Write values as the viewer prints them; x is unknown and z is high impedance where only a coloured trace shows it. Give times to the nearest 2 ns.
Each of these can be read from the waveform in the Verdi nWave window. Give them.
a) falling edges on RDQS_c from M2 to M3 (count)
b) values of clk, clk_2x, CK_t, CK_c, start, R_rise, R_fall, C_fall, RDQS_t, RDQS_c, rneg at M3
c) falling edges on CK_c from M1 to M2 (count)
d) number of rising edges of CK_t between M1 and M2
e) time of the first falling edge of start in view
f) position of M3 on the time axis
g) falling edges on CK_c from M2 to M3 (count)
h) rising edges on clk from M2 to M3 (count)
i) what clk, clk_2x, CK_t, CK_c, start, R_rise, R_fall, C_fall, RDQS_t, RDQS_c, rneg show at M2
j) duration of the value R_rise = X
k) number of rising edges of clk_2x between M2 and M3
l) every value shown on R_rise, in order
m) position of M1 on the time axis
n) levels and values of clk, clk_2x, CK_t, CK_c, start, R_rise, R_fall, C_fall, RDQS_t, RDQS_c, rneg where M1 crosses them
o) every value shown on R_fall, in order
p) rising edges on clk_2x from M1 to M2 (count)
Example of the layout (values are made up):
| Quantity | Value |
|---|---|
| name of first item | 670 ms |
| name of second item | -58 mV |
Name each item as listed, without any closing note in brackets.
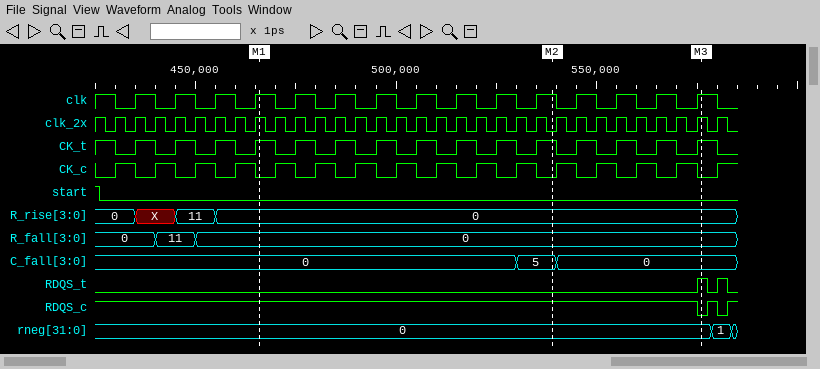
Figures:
| Quantity | Value |
|---|---|
| falling edges on RDQS_c from M2 to M3 | 1 |
| values of clk, clk_2x, CK_t, CK_c, start, R_rise, R_fall, C_fall, RDQS_t, RDQS_c, rneg at M3 | clk=1, clk_2x=1, CK_t=1, CK_c=0, start=0, R_rise=0, R_fall=0, C_fall=0, RDQS_t=1, RDQS_c=0, rneg=0 |
| falling edges on CK_c from M1 to M2 | 7 |
| number of rising edges of CK_t between M1 and M2 | 7 |
| time of the first falling edge of start in view | 426 ns |
| position of M3 on the time axis | 576 ns |
| falling edges on CK_c from M2 to M3 | 4 |
| rising edges on clk from M2 to M3 | 4 |
| what clk, clk_2x, CK_t, CK_c, start, R_rise, R_fall, C_fall, RDQS_t, RDQS_c, rneg show at M2 | clk=1, clk_2x=0, CK_t=1, CK_c=0, start=0, R_rise=0, R_fall=0, C_fall=5, RDQS_t=0, RDQS_c=1, rneg=0 |
| duration of the value R_rise = X | 10 ns |
| number of rising edges of clk_2x between M2 and M3 | 8 |
| every value shown on R_rise, in order | 0, X, 11, 0 |
| position of M1 on the time axis | 466 ns |
| levels and values of clk, clk_2x, CK_t, CK_c, start, R_rise, R_fall, C_fall, RDQS_t, RDQS_c, rneg where M1 crosses them | clk=1, clk_2x=1, CK_t=1, CK_c=0, start=0, R_rise=0, R_fall=0, C_fall=0, RDQS_t=0, RDQS_c=1, rneg=0 |
| every value shown on R_fall, in order | 0, 11, 0 |
| rising edges on clk_2x from M1 to M2 | 14 |
